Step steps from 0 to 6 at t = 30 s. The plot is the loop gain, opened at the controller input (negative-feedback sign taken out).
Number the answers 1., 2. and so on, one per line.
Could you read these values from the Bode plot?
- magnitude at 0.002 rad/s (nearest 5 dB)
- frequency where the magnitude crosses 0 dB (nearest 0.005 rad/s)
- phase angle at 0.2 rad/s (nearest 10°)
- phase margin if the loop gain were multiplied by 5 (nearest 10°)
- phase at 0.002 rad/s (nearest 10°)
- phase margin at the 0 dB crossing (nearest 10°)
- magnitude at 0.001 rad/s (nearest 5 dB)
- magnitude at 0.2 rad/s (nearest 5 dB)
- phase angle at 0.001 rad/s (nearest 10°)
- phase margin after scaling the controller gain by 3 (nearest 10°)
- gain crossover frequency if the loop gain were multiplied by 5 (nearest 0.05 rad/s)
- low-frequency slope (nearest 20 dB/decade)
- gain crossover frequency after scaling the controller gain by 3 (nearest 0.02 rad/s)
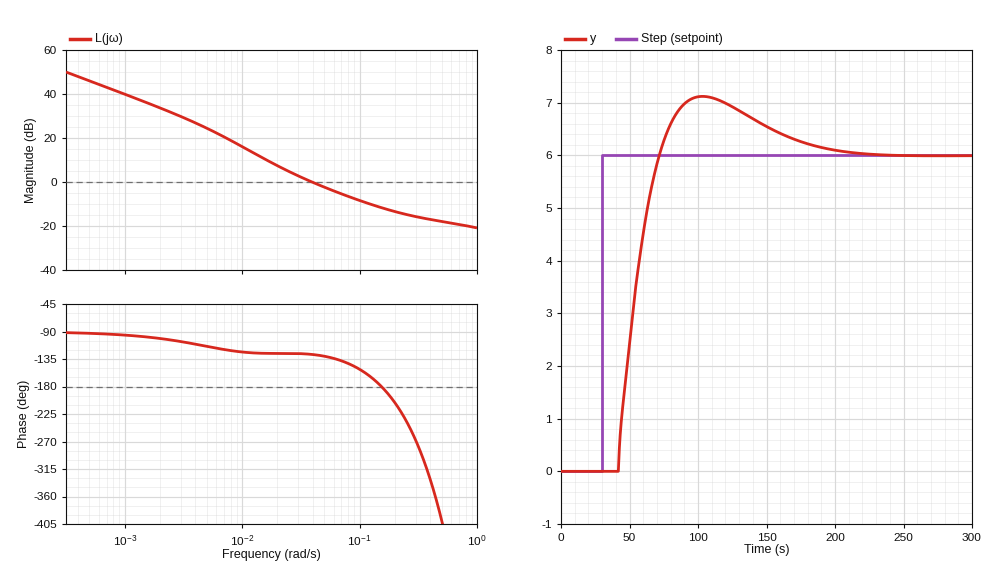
1. 35 dB
2. 0.040 rad/s
3. -210°
4. -40°
5. -100°
6. 50°
7. 40 dB
8. -15 dB
9. -100°
10. 20°
11. 0.20 rad/s
12. -20 dB/decade
13. 0.12 rad/s
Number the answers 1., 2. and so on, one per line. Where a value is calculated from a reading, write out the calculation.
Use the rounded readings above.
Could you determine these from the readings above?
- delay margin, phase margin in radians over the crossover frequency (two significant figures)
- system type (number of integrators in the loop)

1. 50 × π / 180 / 0.04 = 22 s
2. 1
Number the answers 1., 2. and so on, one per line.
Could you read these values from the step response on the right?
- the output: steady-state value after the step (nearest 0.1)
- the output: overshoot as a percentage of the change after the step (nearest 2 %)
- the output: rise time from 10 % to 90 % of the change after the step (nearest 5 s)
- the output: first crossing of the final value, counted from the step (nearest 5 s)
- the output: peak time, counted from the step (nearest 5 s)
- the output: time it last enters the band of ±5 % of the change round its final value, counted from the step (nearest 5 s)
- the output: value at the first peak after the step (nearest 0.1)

1. 6.0
2. 18 %
3. 25 s
4. 40 s
5. 75 s
6. 140 s
7. 7.1
